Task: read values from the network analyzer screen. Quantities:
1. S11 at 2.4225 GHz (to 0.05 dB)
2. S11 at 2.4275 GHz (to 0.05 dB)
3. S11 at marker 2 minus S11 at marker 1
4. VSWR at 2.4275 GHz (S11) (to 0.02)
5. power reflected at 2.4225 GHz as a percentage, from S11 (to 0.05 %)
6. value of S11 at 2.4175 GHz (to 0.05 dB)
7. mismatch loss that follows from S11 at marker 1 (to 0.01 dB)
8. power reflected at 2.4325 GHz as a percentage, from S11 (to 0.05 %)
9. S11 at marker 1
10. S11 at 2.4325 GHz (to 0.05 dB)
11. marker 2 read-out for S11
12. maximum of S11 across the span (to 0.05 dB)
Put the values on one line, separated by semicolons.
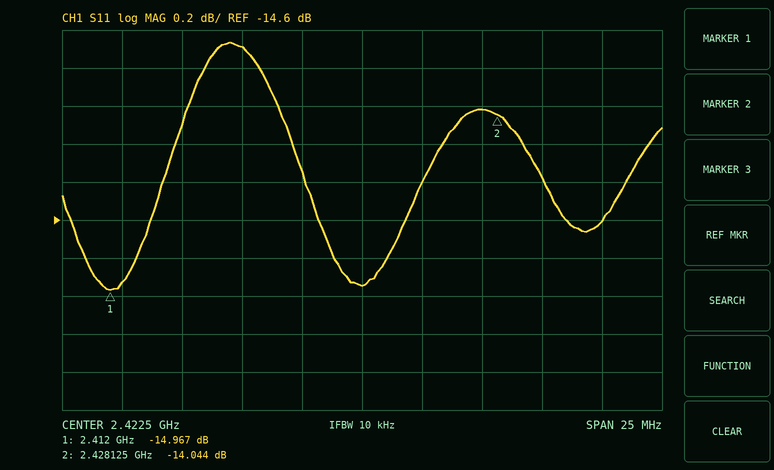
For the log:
-14.95 dB; -14.00 dB; 0.923 dB; 1.50; 3.20 %; -13.70 dB; 0.14 dB; 3.45 %; -14.967 dB; -14.60 dB; -14.044 dB; -13.65 dB
